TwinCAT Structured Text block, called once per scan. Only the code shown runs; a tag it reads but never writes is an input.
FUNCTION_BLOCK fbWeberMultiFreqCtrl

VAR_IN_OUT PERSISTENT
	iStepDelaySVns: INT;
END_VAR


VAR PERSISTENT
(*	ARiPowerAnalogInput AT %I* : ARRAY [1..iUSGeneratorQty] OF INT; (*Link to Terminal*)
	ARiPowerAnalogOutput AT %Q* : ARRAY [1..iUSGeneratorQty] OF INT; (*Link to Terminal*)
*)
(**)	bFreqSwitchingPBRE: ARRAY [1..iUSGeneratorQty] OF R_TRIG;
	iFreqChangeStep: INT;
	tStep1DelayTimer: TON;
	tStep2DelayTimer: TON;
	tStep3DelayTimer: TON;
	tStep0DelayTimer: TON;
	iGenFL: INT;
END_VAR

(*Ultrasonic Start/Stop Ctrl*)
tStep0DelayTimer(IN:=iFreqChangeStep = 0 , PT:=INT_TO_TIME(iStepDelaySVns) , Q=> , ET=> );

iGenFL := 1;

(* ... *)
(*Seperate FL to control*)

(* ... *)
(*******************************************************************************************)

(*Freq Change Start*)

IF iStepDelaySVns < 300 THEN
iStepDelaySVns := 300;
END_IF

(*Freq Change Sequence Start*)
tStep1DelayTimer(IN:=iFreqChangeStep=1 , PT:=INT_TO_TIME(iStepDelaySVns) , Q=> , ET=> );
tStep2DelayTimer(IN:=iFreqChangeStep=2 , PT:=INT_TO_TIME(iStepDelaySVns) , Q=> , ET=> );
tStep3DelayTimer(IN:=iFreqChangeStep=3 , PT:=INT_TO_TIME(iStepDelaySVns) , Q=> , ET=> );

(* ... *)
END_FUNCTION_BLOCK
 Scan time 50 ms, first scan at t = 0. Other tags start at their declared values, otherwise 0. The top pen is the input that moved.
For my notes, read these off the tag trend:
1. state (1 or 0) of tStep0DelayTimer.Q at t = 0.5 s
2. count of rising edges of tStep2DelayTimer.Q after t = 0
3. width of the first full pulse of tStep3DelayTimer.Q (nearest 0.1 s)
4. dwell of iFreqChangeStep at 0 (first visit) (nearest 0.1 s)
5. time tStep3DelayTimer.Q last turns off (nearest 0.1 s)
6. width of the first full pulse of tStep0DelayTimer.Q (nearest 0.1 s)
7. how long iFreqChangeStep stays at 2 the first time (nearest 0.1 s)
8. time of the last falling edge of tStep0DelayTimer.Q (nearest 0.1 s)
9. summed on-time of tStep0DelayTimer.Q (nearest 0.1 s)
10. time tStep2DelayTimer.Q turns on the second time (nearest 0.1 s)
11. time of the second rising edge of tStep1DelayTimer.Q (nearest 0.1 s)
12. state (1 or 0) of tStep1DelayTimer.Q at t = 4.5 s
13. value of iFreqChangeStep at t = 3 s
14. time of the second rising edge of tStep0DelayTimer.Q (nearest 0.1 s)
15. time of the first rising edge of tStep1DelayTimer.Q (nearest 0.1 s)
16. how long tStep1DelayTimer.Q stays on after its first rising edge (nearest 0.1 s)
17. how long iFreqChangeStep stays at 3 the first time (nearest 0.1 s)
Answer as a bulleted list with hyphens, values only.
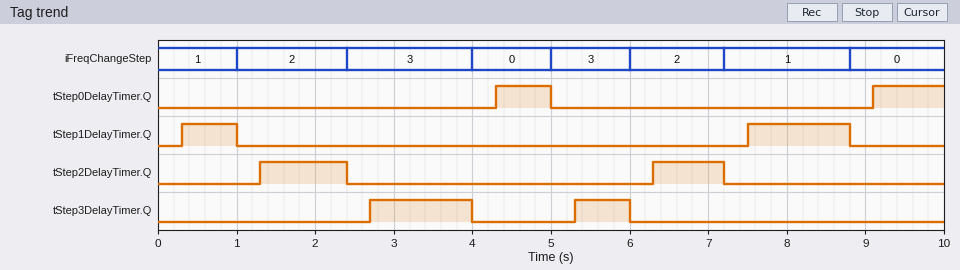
- 0
- 2
- 1.3 s
- 1.0 s
- 6.0 s
- 0.7 s
- 1.4 s
- 5.0 s
- 1.6 s
- 6.3 s
- 7.5 s
- 0
- 3
- 9.1 s
- 0.3 s
- 0.7 s
- 1.6 s
